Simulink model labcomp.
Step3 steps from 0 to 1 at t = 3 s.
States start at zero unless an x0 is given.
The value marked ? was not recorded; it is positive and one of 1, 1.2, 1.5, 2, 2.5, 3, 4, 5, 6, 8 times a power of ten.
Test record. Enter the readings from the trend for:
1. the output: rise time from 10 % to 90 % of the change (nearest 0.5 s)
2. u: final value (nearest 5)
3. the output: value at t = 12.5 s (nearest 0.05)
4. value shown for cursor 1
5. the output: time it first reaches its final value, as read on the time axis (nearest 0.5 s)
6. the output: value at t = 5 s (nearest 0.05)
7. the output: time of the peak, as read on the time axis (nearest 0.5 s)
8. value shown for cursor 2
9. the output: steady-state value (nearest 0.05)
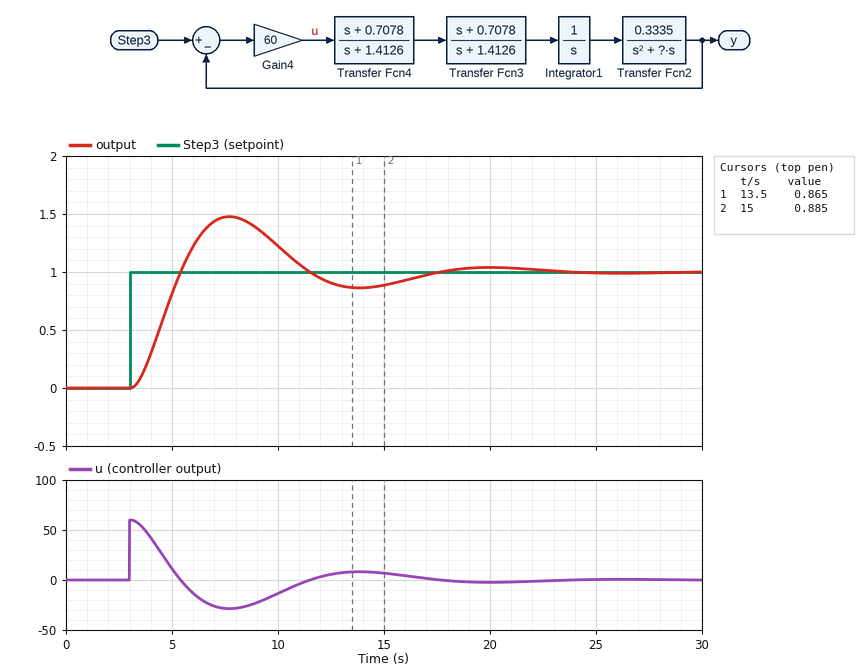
1.5 s
0
0.90
0.865
5.5 s
0.80
7.5 s
0.885
1.00
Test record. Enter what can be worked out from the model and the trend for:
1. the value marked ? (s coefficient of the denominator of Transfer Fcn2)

20
